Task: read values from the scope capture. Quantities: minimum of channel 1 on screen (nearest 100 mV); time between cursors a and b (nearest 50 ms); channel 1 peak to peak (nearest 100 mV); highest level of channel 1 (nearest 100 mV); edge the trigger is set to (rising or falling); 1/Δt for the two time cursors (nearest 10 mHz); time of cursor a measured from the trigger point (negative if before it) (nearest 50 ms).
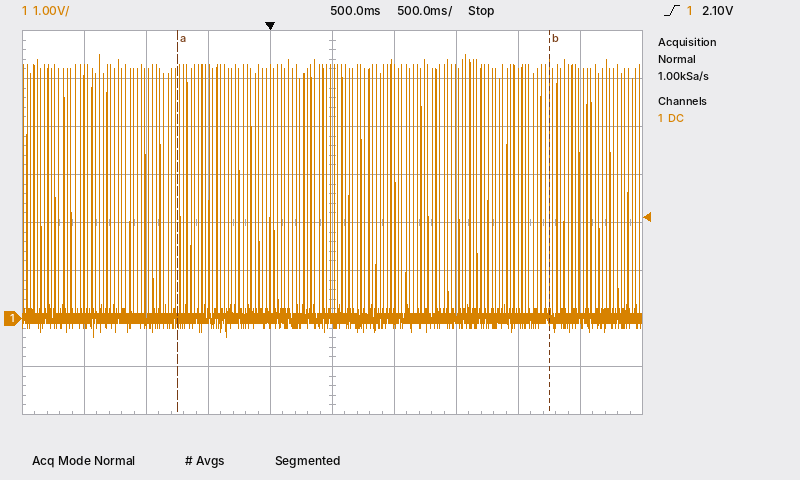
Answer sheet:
-400 mV
3.00 s
5.9 V
5.5 V
rising
330 mHz
-750 ms
